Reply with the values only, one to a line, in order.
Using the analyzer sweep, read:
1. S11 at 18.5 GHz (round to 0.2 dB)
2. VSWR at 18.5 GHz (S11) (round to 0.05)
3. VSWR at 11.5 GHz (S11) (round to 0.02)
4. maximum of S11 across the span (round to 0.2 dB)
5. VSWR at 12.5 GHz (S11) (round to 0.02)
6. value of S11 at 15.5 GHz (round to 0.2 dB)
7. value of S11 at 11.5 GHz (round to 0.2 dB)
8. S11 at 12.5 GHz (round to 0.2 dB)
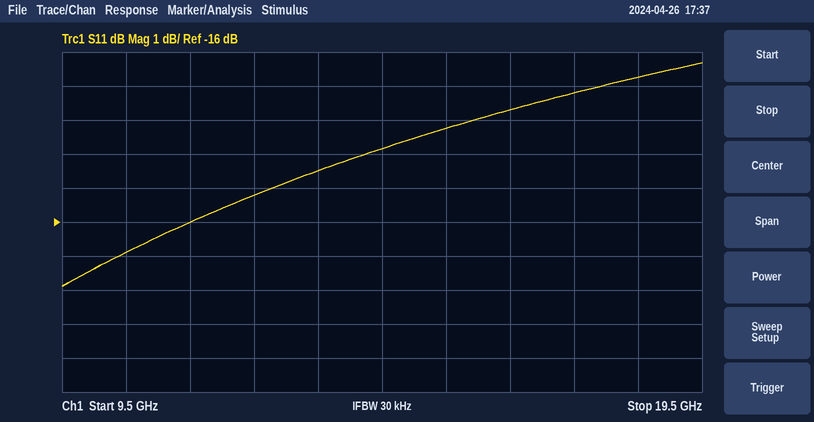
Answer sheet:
-11.8 dB
1.70
1.38
-11.4 dB
1.42
-13.2 dB
-16.0 dB
-15.2 dB
